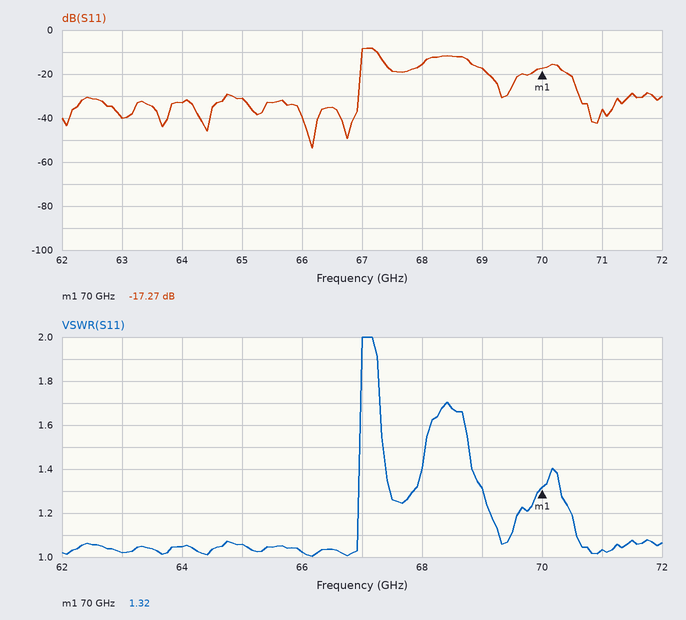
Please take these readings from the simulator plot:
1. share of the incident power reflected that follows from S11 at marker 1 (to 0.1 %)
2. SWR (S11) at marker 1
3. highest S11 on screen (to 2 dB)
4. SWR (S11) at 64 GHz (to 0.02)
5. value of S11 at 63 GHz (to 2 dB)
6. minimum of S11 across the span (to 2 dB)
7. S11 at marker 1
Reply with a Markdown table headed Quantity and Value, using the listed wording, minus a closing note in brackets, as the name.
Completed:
| Quantity | Value |
|---|---|
| share of the incident power reflected that follows from S11 at marker 1 | 1.9 % |
| SWR (S11) at marker 1 | 1.32 |
| highest S11 on screen | -8 dB |
| SWR (S11) at 64 GHz | 1.04 |
| value of S11 at 63 GHz | -40 dB |
| minimum of S11 across the span | -54 dB |
| S11 at marker 1 | -17.27 dB |
